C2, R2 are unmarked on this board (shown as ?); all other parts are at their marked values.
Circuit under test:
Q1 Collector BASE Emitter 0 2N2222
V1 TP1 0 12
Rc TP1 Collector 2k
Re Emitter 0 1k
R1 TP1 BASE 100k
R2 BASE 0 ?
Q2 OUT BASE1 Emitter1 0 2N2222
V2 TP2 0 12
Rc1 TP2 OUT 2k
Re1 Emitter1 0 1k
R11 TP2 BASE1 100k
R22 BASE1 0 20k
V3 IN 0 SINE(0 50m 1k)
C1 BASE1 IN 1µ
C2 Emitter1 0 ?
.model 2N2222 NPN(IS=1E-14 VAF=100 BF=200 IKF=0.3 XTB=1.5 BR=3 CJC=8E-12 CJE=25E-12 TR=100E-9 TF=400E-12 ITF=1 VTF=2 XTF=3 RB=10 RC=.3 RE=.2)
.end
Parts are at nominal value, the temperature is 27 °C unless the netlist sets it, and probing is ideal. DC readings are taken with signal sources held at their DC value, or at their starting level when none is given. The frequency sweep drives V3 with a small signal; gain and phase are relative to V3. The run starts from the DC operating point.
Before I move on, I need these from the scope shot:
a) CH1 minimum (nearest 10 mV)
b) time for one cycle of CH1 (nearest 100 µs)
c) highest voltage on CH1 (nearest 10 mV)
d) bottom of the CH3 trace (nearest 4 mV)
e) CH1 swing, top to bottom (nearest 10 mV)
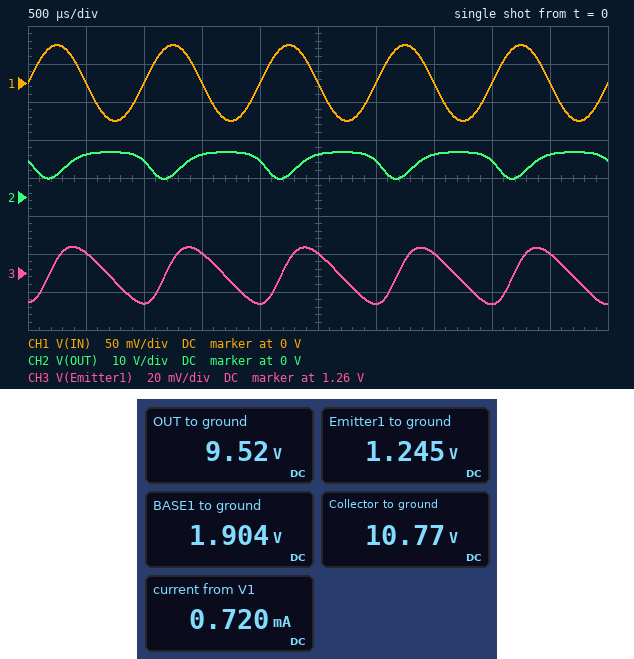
-50 mV
1.0 ms
50 mV
1.244 V
100 mV
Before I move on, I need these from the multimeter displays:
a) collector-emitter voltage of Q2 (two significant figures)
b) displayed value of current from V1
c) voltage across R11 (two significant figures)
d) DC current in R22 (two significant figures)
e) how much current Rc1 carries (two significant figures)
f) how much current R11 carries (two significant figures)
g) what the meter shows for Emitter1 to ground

8.3 V
0.720 mA
10 V
95 µA
1.2 mA
100 µA
1.245 V
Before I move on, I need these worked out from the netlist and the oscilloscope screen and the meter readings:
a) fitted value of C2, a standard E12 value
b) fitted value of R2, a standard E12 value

18 µF
12 kΩ
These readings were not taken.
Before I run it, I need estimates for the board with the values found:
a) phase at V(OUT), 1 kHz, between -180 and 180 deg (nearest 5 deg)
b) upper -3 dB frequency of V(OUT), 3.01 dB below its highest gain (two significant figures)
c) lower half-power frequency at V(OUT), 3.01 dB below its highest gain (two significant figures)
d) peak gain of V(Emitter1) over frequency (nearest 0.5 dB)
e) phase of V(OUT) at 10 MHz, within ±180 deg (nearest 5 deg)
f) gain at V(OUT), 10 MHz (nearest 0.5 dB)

-155 deg
15 MHz
450 Hz
-1.0 dB
145 deg
37.5 dB
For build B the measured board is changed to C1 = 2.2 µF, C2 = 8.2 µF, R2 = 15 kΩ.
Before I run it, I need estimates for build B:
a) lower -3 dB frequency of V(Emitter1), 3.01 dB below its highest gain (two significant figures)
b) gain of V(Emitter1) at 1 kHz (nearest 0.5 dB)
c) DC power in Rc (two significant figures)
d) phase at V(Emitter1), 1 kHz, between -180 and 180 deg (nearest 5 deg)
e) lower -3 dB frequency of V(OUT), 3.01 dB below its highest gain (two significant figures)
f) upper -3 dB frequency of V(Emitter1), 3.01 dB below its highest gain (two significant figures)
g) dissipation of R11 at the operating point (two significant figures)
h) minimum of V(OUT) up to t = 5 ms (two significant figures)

4.6 Hz
-3.5 dB
1.5 mW
-45 deg
930 Hz
940 Hz
1.0 mW
5.7 V
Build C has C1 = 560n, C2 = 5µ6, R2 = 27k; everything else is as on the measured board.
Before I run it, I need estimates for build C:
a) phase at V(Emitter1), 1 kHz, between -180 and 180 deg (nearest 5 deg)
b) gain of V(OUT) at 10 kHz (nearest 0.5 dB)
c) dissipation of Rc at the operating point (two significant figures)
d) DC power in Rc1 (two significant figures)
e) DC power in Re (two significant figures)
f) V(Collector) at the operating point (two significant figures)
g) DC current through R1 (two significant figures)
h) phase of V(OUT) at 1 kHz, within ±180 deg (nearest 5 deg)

-35 deg
39.0 dB
5.8 mW
3.1 mW
2.9 mW
8.6 V
96 µA
-125 deg
